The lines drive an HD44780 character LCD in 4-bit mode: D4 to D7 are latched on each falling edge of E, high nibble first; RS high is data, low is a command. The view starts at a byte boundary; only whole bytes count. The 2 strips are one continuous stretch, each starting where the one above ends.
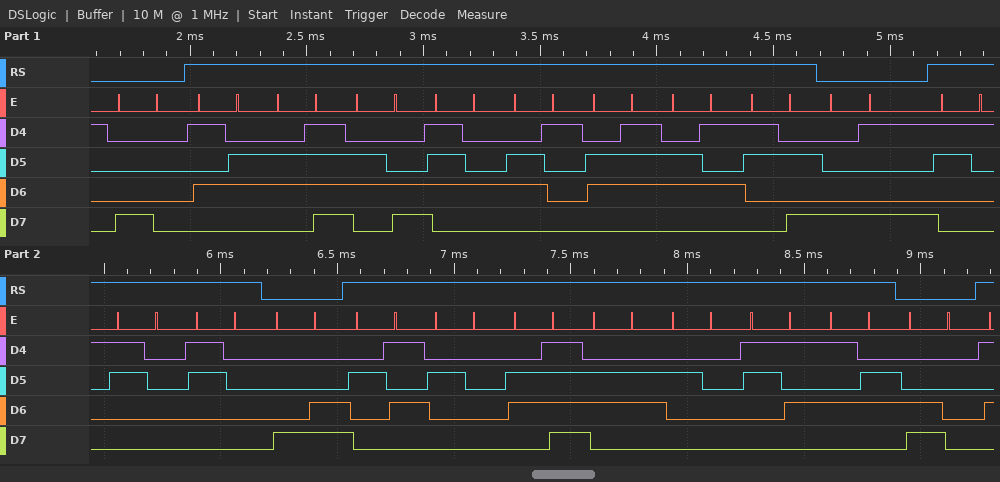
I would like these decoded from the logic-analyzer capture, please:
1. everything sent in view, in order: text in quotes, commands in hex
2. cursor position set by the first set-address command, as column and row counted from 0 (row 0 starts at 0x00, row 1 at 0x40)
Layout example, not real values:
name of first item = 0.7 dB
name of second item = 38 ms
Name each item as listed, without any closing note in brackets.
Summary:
everything sent in view, in order: text in quotes, commands in hex = 0x80 "Voltage:" 0x89 "100" 0x8C "% of 5V" 0xC0
cursor position set by the first set-address command, as column and row counted from 0 = column 0, row 0
